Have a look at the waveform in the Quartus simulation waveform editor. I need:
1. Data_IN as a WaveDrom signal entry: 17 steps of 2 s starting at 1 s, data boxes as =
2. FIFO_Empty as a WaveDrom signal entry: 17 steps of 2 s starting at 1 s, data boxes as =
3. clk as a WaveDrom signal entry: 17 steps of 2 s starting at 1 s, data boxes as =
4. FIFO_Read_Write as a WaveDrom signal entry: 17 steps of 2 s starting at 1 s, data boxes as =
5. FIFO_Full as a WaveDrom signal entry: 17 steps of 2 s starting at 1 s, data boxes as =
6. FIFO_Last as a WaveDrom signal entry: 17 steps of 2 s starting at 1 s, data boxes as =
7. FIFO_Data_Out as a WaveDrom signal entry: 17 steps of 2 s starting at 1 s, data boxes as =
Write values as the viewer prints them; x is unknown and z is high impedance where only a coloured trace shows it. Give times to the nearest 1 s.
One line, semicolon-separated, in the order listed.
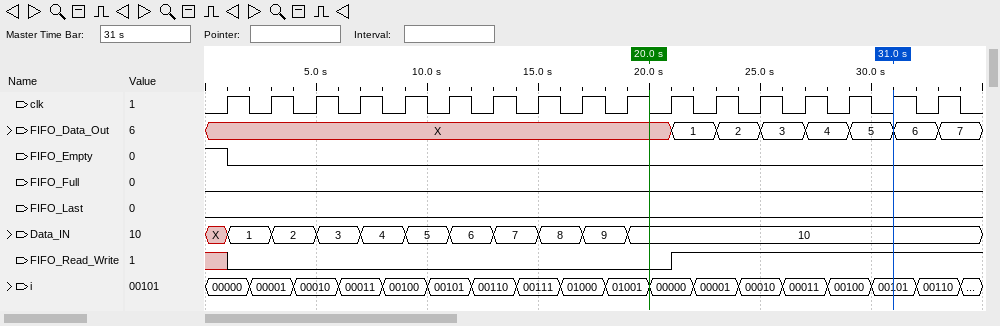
{name: 'Data_IN', wave: '==========.......', data: '1 2 3 4 5 6 7 8 9 10'}; {name: 'FIFO_Empty', wave: '0................'}; {name: 'clk', wave: 'p................'}; {name: 'FIFO_Read_Write', wave: '0.........1......'}; {name: 'FIFO_Full', wave: '0................'}; {name: 'FIFO_Last', wave: '0................'}; {name: 'FIFO_Data_Out', wave: 'x.........=======', data: '1 2 3 4 5 6 7'}
